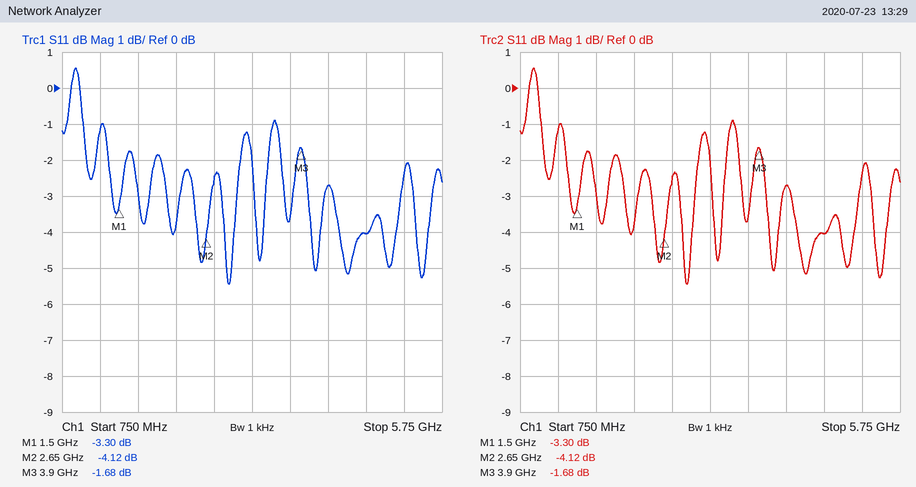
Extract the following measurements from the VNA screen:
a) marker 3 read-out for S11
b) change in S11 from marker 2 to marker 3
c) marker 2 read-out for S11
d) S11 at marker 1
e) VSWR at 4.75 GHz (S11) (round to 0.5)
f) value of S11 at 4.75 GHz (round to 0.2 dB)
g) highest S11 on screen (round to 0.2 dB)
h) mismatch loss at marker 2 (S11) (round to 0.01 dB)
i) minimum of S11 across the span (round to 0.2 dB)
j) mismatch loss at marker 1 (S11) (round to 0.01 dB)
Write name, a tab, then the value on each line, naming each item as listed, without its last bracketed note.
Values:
marker 3 read-out for S11	-1.68 dB
change in S11 from marker 2 to marker 3	2.44 dB
marker 2 read-out for S11	-4.12 dB
S11 at marker 1	-3.30 dB
VSWR at 4.75 GHz (S11)	4.5
value of S11 at 4.75 GHz	-4.0 dB
highest S11 on screen	0.6 dB
mismatch loss at marker 2 (S11)	2.13 dB
minimum of S11 across the span	-5.4 dB
mismatch loss at marker 1 (S11)	2.74 dB
